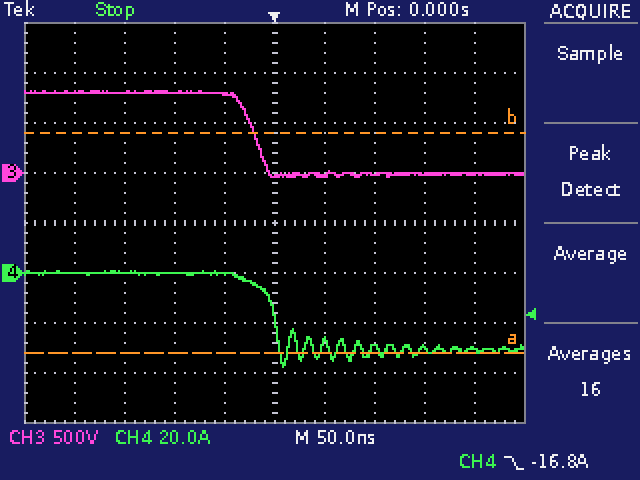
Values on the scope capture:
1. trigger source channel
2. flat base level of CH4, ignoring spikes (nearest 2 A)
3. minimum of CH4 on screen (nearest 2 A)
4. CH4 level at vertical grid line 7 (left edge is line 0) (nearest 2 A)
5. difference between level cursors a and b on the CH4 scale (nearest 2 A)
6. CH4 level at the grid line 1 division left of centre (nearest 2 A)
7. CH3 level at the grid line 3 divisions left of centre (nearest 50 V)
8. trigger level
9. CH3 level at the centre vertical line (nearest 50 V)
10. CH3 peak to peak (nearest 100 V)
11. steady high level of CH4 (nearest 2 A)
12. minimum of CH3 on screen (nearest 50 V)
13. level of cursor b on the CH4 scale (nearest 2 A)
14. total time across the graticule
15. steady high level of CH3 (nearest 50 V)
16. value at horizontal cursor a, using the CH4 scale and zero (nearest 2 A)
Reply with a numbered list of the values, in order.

1. CH4
2. -30 A
3. -38 A
4. -30 A
5. 88 A
6. 0 A
7. 800 V
8. -16.8 A
9. -50 V
10. 900 V
11. 0 A
12. -50 V
13. 56 A
14. 500 ns
15. 800 V
16. -32 A
